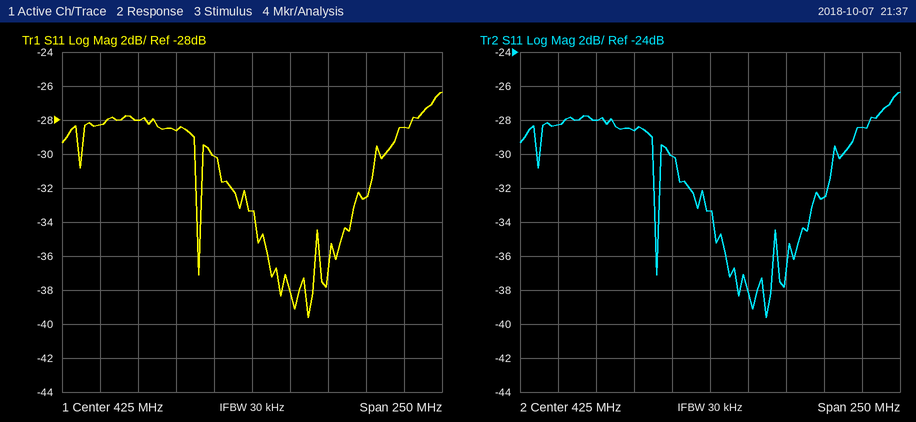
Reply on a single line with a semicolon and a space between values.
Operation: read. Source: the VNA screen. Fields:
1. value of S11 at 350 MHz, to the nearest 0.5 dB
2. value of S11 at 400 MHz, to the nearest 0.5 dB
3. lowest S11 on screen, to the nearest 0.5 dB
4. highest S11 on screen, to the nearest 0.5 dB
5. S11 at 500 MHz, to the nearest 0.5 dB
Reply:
-28.0 dB; -30.0 dB; -39.5 dB; -26.5 dB; -32.5 dB
